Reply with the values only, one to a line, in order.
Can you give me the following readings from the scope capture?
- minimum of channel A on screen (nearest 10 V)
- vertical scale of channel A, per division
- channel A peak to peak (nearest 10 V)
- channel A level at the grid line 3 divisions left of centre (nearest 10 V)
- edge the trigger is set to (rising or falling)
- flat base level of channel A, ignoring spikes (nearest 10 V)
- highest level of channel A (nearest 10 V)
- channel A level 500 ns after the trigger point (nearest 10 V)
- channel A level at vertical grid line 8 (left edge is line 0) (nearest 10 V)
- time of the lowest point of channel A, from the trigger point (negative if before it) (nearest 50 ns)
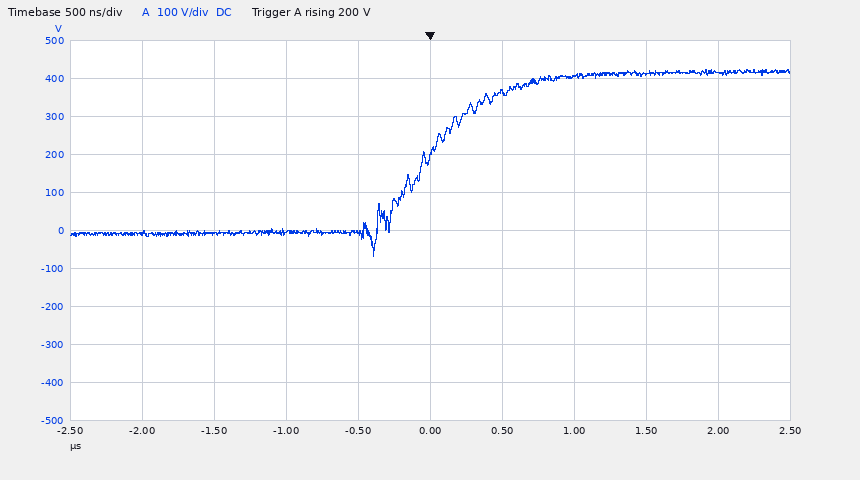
-70 V
100 V
490 V
-10 V
rising
-10 V
420 V
360 V
410 V
-400 ns
